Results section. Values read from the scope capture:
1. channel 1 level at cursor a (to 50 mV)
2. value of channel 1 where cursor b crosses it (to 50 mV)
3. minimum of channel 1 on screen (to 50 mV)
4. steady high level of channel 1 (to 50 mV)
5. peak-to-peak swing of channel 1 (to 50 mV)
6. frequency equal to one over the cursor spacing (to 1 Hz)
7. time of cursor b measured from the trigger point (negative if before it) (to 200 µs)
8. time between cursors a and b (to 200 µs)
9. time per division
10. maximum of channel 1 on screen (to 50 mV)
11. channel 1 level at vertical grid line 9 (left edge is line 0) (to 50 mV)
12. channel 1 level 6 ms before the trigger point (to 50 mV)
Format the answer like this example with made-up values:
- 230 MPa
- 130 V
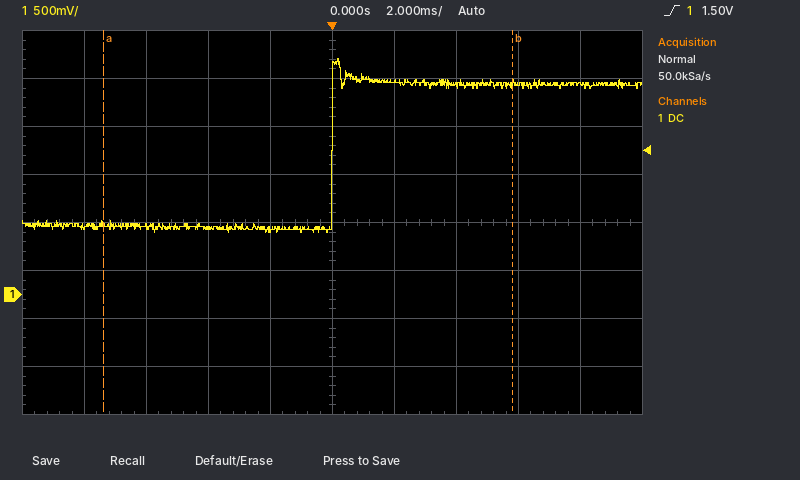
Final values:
- 750 mV
- 2.20 V
- 650 mV
- 2.20 V
- 1.80 V
- 76 Hz
- +5.8 ms
- 13.2 ms
- 2 ms
- 2.45 V
- 2.20 V
- 700 mV
